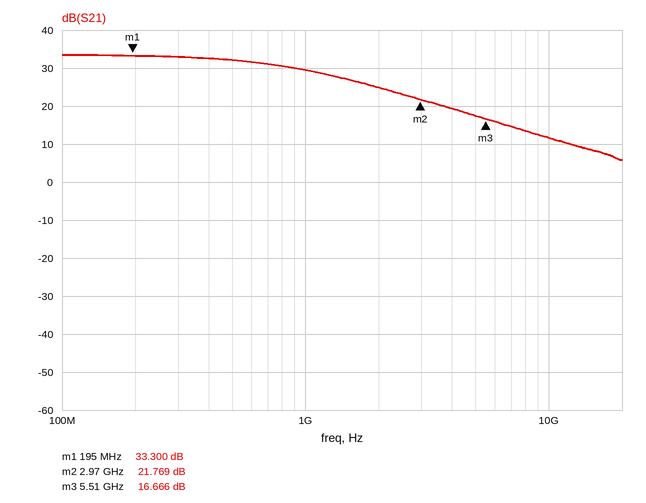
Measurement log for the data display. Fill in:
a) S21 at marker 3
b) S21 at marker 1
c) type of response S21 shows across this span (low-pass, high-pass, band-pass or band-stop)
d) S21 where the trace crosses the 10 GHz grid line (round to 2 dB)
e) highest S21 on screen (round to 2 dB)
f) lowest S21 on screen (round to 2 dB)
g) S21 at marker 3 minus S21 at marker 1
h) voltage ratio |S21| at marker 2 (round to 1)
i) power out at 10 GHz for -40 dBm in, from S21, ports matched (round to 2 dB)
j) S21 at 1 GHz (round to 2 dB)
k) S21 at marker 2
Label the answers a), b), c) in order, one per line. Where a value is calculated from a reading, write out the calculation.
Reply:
a) 16.666 dB
b) 33.300 dB
c) low-pass
d) 12 dB
e) 34 dB
f) 6 dB
g) 16.666 − (33.3) = -16.634 dB
h) 10^(21.769/20) ≈ 12
i) -40 dBm + (12 dB) = -28 dBm
j) 30 dB
k) 21.769 dB
